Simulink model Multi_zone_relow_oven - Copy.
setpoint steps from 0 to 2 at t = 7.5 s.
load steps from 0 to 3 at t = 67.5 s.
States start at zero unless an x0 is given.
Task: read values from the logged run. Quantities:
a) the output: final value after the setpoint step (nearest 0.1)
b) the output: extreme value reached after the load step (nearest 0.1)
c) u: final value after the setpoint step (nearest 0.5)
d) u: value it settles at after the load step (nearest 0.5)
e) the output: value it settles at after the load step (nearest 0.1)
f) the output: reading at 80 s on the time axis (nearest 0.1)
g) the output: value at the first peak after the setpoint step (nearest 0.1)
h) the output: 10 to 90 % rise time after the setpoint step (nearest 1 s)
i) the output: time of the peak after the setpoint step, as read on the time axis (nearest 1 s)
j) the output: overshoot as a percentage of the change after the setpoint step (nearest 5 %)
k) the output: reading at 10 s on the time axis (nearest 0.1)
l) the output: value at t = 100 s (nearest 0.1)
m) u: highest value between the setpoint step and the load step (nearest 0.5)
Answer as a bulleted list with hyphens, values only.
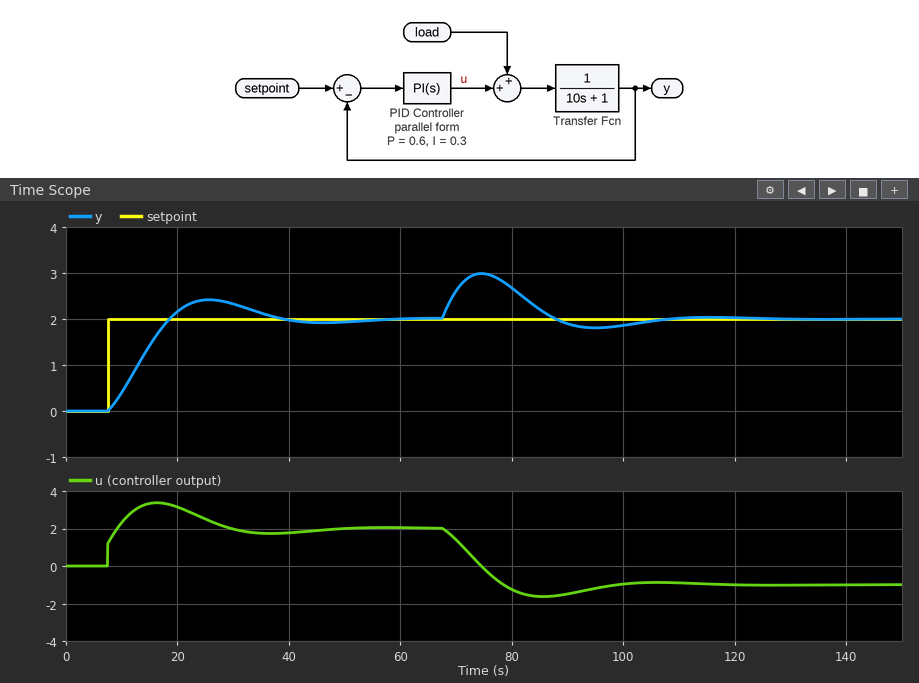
- 2.0
- 3.0
- 2.0
- -1.0
- 2.0
- 2.7
- 2.4
- 8 s
- 26 s
- 20 %
- 0.4
- 1.9
- 3.5
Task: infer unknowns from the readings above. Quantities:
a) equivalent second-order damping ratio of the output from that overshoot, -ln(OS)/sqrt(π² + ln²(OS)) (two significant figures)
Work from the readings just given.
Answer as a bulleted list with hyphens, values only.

- 0.46
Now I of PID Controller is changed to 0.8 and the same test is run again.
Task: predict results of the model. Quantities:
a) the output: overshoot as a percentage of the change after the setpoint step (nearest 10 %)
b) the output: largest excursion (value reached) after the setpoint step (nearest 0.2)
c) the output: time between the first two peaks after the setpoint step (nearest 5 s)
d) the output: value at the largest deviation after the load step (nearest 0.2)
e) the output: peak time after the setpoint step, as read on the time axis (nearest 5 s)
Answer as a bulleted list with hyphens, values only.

- 40 %
- 2.8
- 25 s
- 2.8
- 20 s
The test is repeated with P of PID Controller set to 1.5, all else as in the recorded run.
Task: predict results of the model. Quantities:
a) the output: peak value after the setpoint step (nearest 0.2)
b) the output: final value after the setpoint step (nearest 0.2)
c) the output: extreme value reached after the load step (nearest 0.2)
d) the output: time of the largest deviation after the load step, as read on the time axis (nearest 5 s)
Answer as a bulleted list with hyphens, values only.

- 2.2
- 2.0
- 2.8
- 75 s
